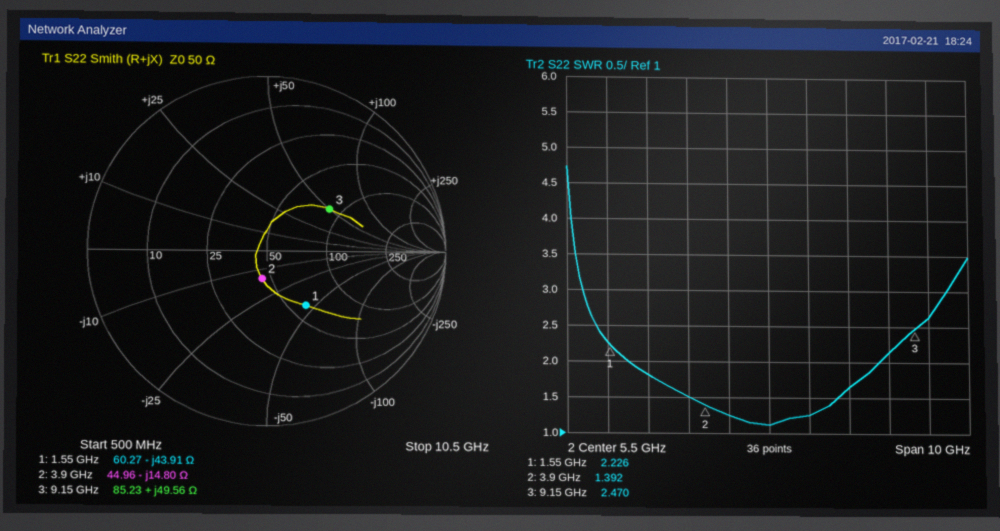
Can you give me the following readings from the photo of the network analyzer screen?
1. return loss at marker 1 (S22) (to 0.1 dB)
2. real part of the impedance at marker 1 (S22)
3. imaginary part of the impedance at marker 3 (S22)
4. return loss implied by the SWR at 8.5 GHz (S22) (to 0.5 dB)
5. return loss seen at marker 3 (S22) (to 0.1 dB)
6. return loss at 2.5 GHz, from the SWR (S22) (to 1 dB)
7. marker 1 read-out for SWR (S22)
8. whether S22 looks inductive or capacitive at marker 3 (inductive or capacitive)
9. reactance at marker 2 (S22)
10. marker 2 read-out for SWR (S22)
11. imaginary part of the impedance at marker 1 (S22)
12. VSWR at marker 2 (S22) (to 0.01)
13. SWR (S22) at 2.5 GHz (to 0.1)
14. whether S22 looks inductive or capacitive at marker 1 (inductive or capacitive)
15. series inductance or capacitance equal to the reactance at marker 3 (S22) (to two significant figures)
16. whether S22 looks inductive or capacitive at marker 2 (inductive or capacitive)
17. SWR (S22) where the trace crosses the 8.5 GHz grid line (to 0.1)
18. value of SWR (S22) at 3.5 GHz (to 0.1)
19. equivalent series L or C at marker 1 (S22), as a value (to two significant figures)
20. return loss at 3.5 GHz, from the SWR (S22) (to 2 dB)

8.4 dB
60.27 Ω
+49.56 Ω
9.0 dB
7.5 dB
11 dB
2.226
inductive
-14.80 Ω
1.392
-43.91 Ω
1.39
1.8
capacitive
860 pH
capacitive
2.1
1.5
2.3 pF
14 dB
